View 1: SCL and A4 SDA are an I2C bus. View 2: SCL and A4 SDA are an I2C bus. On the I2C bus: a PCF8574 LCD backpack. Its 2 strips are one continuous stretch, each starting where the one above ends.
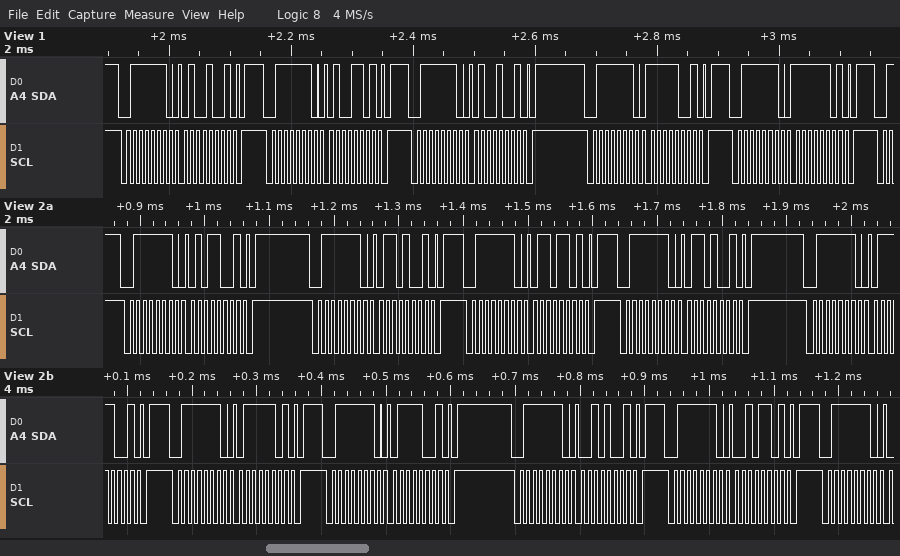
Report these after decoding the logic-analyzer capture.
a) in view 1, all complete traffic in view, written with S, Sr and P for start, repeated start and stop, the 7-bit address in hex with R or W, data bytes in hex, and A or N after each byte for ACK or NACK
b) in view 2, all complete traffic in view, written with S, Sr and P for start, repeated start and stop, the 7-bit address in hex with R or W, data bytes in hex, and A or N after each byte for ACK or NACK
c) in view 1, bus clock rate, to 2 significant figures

S 3FW A 49 A P S 3FW A 4D A P S 3FW A 49 A P S 3FW A F9 A P S 3FW A FD A P
S 3FW A 59 A P S 3FW A 69 A P S 3FW A 6D A P S 3FW A 69 A P S 3FW A 79 A P S 3FW A 7D A P S 3FW A 79 A P S 3FW A 29 A P S 3FW A 2D A P S 3FW A
100 kHz
